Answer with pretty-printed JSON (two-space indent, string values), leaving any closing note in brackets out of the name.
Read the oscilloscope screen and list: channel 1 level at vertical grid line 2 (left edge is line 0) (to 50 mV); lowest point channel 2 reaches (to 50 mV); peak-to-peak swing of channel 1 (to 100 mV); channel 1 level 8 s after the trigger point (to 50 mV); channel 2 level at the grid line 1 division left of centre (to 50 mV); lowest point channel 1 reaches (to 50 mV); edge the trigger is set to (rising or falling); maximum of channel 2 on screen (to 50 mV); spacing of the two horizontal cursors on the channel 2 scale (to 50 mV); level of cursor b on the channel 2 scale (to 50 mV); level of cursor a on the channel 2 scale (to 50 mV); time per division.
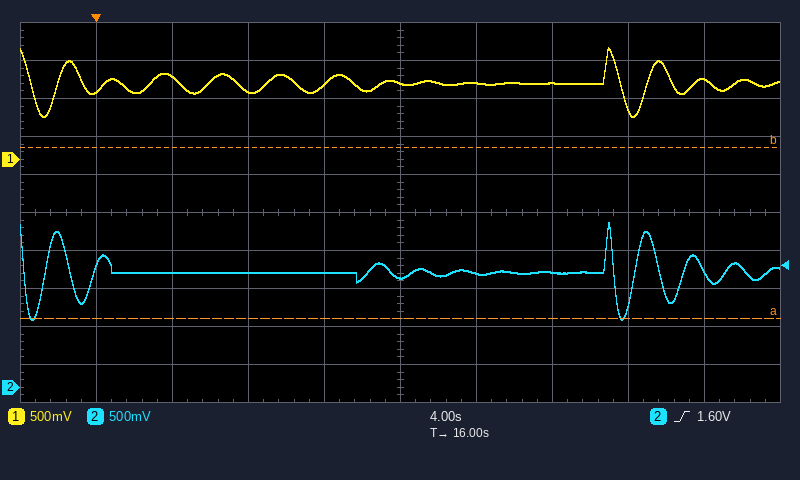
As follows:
{
  "channel 1 level at vertical grid line 2 (left edge is line 0)": "1.10 V",
  "lowest point channel 2 reaches": "900 mV",
  "peak-to-peak swing of channel 1": "900 mV",
  "channel 1 level 8 s after the trigger point": "900 mV",
  "channel 2 level at the grid line 1 division left of centre": "1.50 V",
  "lowest point channel 1 reaches": "550 mV",
  "edge the trigger is set to": "rising",
  "maximum of channel 2 on screen": "2.15 V",
  "spacing of the two horizontal cursors on the channel 2 scale": "2.25 V",
  "level of cursor b on the channel 2 scale": "3.15 V",
  "level of cursor a on the channel 2 scale": "900 mV",
  "time per division": "4 s"
}
